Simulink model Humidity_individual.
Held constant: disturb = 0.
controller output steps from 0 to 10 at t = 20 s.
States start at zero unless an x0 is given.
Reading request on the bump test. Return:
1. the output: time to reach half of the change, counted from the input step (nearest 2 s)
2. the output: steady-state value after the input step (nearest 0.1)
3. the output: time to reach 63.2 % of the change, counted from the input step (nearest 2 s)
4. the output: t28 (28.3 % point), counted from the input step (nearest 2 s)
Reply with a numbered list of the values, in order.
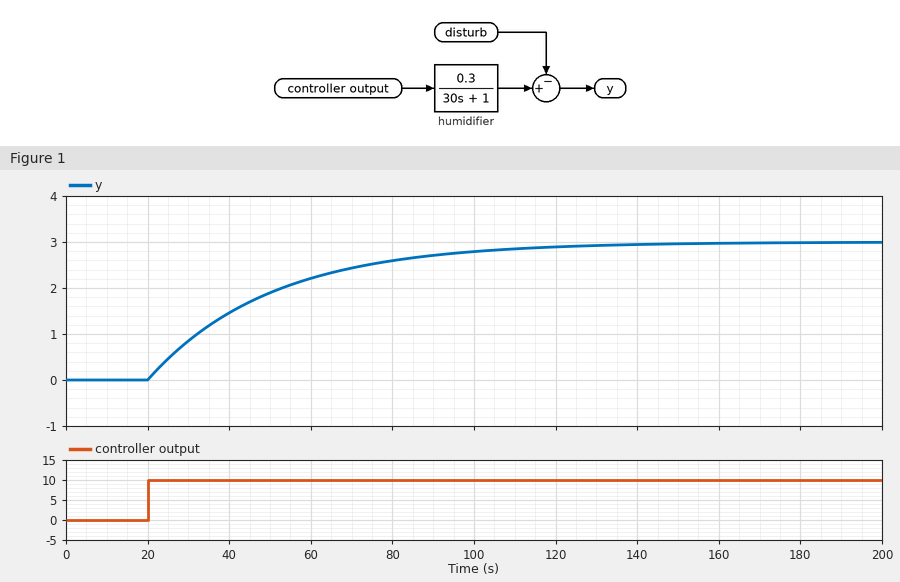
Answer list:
1. 20 s
2. 3.0
3. 30 s
4. 10 s
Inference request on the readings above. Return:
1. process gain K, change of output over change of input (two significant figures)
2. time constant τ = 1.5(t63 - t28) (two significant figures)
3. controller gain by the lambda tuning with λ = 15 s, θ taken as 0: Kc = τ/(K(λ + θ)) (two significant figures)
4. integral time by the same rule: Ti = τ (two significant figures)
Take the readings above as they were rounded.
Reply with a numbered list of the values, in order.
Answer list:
1. 0.30
2. 30 s
3. 6.7
4. 30 s
